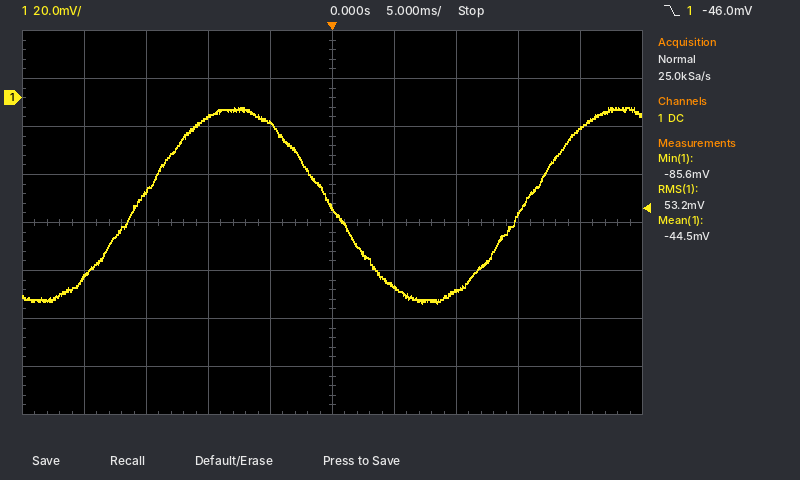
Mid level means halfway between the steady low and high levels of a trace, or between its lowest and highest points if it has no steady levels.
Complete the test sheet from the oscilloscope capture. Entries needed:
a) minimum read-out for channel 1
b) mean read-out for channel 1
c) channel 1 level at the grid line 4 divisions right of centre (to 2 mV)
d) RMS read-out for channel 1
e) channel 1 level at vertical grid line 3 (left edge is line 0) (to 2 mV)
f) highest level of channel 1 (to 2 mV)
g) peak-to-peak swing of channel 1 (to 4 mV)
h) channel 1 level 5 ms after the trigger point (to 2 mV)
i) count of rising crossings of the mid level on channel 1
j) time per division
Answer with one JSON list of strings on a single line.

["-85.6 mV", "-44.5 mV", "-14 mV", "53.2 mV", "-8 mV", "-4 mV", "80 mV", "-78 mV", "2", "5 ms"]
